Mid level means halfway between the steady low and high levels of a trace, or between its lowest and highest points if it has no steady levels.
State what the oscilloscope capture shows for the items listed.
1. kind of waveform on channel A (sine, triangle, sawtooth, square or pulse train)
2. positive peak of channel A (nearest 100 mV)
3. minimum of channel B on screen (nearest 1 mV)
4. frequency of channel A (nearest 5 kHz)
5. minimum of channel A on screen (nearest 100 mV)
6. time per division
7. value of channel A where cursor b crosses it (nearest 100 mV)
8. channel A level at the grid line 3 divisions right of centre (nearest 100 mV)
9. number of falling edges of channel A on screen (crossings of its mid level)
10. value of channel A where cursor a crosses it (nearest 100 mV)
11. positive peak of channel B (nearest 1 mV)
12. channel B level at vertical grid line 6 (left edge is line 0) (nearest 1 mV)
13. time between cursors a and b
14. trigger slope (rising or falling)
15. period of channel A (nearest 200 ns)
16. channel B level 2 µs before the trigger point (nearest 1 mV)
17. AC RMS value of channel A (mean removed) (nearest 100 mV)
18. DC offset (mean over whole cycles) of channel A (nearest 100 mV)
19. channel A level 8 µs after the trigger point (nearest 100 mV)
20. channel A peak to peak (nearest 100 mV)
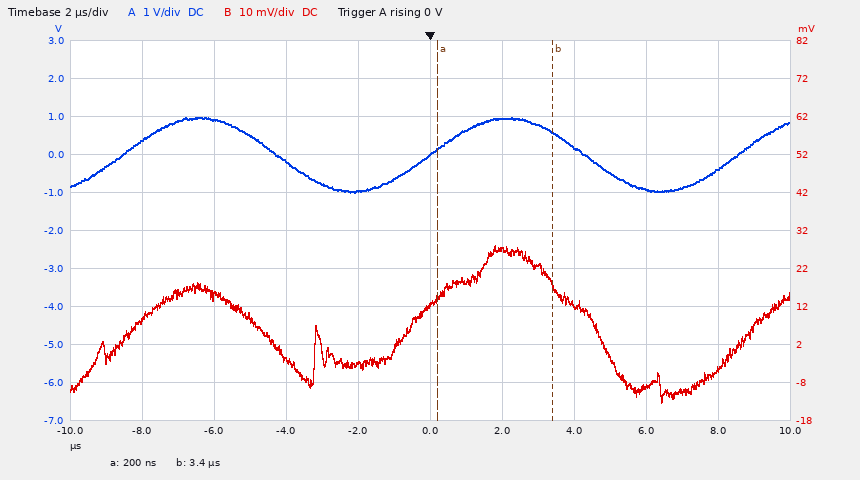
sine
1.0 V
-13 mV
115 kHz
-1.0 V
2 µs
600 mV
-900 mV
2
100 mV
28 mV
27 mV
3.2 µs
rising
8.6 µs
-3 mV
700 mV
0.0 V
-400 mV
2.0 V
